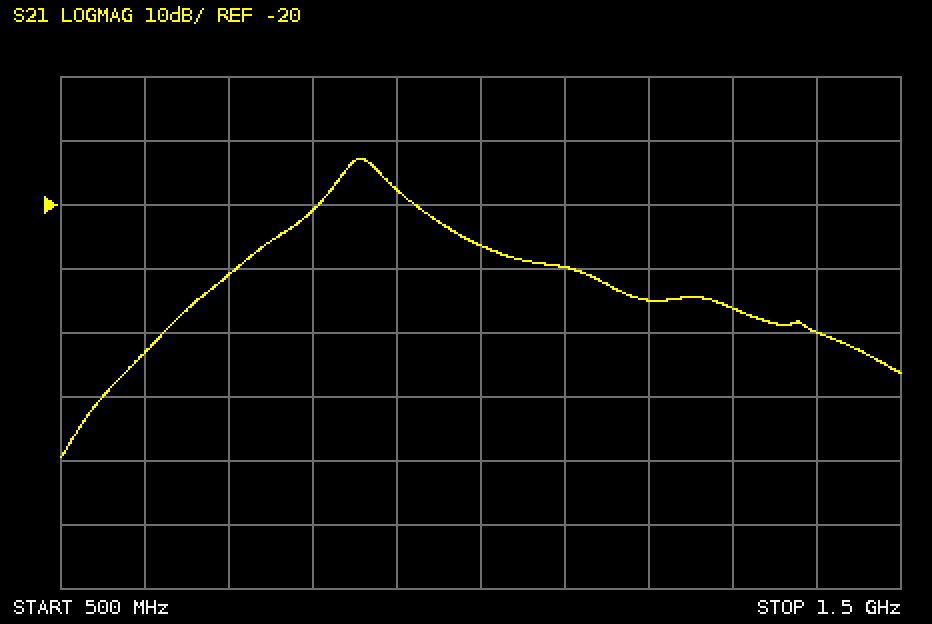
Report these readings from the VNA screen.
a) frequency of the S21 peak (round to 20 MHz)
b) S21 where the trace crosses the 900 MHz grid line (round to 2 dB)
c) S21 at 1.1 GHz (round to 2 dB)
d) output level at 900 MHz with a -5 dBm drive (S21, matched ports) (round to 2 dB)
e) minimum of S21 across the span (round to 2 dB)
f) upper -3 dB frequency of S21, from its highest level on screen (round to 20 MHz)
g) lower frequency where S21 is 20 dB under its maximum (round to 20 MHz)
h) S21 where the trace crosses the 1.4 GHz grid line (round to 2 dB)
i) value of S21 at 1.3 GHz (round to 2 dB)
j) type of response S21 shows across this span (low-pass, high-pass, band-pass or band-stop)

860 MHz
-18 dB
-30 dB
-22 dBm
-60 dB
880 MHz
680 MHz
-40 dB
-36 dB
band-pass
